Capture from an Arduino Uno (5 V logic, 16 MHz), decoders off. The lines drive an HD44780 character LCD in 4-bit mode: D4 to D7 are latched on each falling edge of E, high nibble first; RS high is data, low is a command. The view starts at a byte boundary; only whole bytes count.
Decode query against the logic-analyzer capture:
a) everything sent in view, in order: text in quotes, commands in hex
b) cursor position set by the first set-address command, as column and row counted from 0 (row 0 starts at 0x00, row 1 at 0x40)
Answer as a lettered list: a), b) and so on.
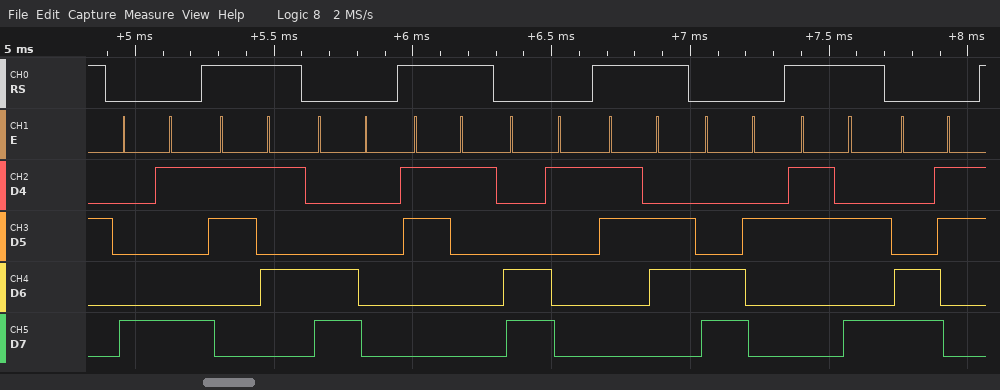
a) 0x89 "5" 0xC0 "1" 0xC1 "6" 0xC2 ":" 0xC3
b) column 9, row 0
